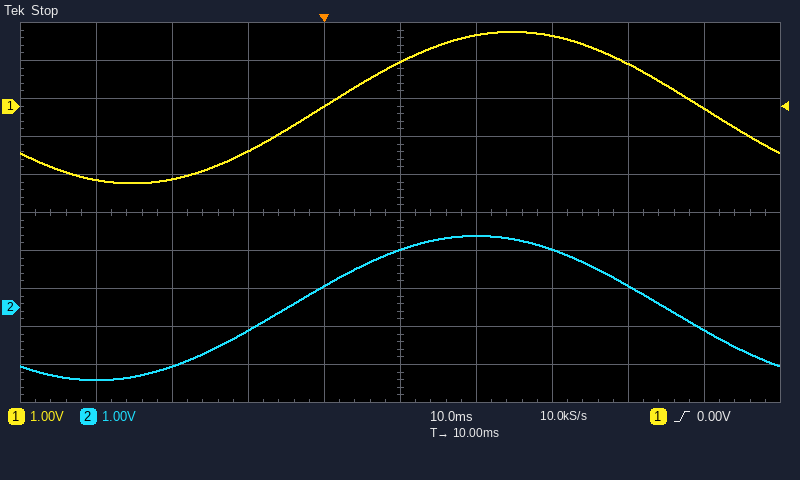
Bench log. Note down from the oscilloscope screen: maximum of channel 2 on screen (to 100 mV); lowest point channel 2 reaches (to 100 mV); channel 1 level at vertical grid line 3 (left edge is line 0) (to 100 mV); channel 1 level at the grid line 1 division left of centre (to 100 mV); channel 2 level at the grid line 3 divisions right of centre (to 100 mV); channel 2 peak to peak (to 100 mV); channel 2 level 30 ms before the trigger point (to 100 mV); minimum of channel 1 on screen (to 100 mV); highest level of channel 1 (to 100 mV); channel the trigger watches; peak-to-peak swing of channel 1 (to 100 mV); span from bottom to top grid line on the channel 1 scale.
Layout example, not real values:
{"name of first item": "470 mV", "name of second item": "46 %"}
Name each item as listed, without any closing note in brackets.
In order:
{"maximum of channel 2 on screen": "1.9 V", "lowest point channel 2 reaches": "-1.9 V", "channel 1 level at vertical grid line 3 (left edge is line 0)": "-1.2 V", "channel 1 level at the grid line 1 division left of centre": "0.0 V", "channel 2 level at the grid line 3 divisions right of centre": "600 mV", "channel 2 peak to peak": "3.8 V", "channel 2 level 30 ms before the trigger point": "-1.9 V", "minimum of channel 1 on screen": "-2.0 V", "highest level of channel 1": "2.0 V", "channel the trigger watches": "channel 1", "peak-to-peak swing of channel 1": "4.0 V", "span from bottom to top grid line on the channel 1 scale": "10 V"}
